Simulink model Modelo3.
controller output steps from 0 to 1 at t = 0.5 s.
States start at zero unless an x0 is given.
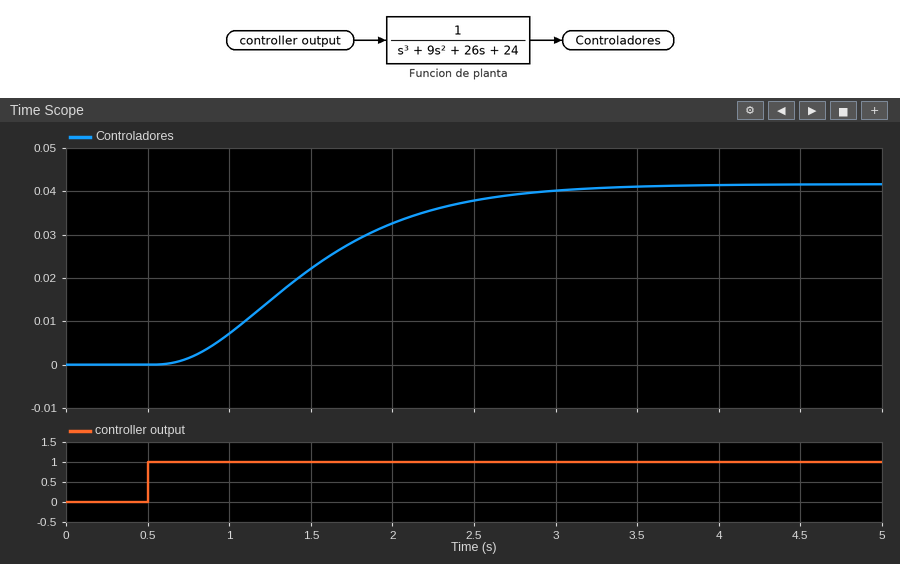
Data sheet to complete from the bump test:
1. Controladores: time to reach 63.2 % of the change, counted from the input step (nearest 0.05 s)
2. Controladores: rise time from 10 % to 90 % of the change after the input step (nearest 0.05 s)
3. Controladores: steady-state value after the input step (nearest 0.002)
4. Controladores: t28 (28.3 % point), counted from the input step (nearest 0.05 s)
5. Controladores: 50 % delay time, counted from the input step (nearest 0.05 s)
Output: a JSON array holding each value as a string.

["1.15 s", "1.55 s", "0.042", "0.65 s", "0.95 s"]
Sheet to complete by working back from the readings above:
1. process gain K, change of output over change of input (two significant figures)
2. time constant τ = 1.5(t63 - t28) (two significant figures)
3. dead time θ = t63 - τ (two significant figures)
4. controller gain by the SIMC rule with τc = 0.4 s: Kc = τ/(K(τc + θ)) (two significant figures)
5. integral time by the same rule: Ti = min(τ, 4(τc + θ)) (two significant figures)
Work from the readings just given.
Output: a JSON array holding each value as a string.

["0.042", "0.75 s", "0.40 s", "22", "0.75 s"]
